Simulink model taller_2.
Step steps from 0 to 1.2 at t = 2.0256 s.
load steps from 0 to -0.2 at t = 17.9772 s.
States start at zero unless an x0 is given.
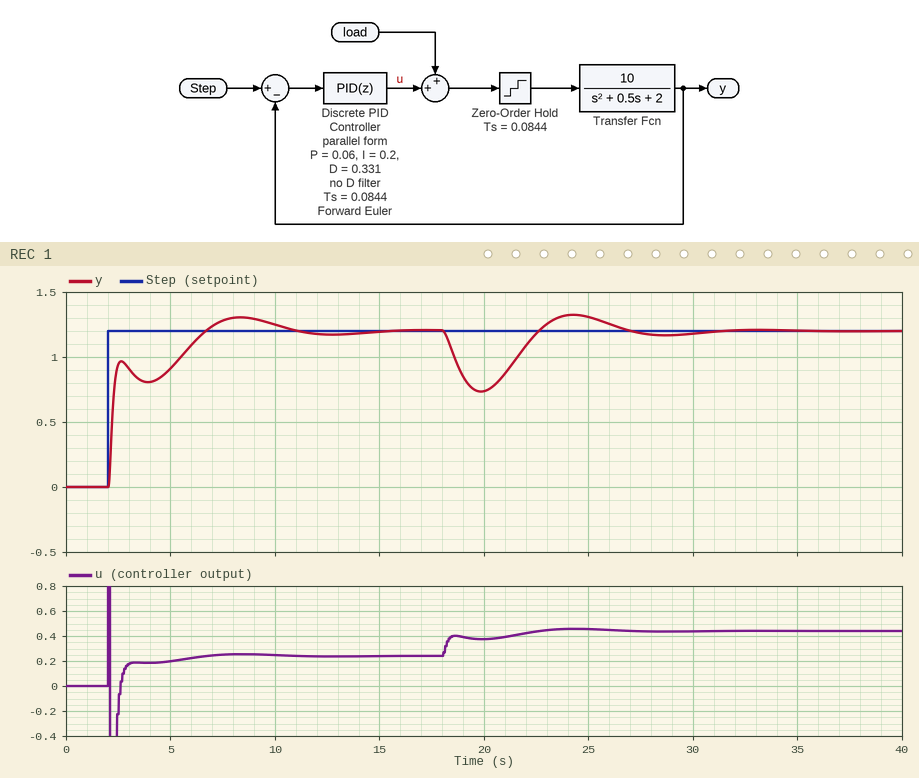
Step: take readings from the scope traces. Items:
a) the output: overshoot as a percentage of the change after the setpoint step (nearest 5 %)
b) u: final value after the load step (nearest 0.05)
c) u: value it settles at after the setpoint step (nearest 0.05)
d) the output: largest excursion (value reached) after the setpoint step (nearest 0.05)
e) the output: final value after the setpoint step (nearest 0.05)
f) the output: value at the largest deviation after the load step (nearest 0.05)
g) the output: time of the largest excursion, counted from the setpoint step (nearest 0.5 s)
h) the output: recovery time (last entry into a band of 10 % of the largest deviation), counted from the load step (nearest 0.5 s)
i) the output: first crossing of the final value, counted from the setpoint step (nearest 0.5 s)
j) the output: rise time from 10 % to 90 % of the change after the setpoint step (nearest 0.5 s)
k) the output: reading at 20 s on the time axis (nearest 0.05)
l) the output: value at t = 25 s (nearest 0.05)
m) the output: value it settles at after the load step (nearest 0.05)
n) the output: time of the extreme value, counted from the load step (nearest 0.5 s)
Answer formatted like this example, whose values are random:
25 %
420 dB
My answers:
10 %
0.45
0.25
1.30
1.20
0.75
6.5 s
8.0 s
4.5 s
4.0 s
0.75
1.30
1.20
2.0 s
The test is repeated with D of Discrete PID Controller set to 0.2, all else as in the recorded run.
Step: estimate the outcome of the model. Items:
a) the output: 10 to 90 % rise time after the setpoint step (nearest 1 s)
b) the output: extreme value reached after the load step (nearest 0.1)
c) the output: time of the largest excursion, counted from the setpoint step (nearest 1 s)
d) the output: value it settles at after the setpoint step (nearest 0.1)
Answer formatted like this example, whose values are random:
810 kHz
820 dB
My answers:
3 s
0.6
5 s
1.2
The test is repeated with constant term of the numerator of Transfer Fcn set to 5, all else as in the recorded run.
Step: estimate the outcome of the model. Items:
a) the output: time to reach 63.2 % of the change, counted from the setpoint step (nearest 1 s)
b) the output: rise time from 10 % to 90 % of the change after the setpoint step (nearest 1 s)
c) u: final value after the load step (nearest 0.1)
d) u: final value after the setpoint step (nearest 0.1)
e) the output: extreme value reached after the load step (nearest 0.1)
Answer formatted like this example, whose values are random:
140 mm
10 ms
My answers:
3 s
5 s
0.7
0.5
0.8
